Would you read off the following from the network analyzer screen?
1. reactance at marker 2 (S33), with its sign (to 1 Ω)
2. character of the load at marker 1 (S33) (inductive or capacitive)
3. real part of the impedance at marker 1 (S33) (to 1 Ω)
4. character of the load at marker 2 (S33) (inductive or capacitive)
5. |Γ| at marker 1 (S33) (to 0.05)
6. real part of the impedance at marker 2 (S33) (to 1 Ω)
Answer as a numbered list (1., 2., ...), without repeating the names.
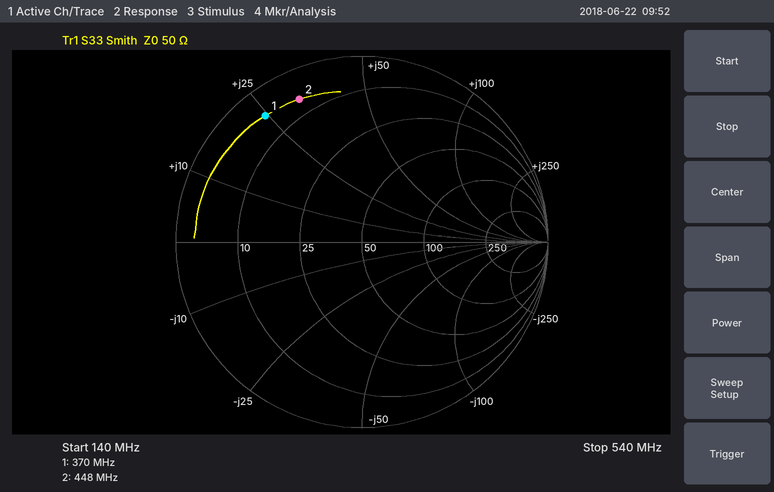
1. +32 Ω
2. inductive
3. 5 Ω
4. inductive
5. 0.85
6. 6 Ω
